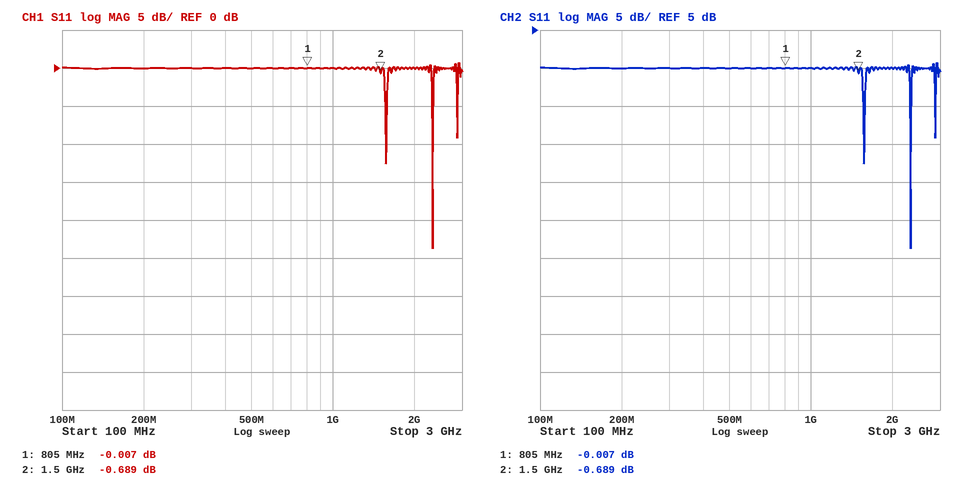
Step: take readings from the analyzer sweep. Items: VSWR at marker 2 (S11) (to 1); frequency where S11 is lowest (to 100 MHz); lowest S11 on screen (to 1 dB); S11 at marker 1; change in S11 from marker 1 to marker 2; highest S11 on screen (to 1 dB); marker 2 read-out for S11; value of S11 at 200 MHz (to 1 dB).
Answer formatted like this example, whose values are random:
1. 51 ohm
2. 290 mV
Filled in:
1. 25
2. 2.3 GHz
3. -24 dB
4. -0.007 dB
5. -0.682 dB
6. 1 dB
7. -0.689 dB
8. 0 dB
